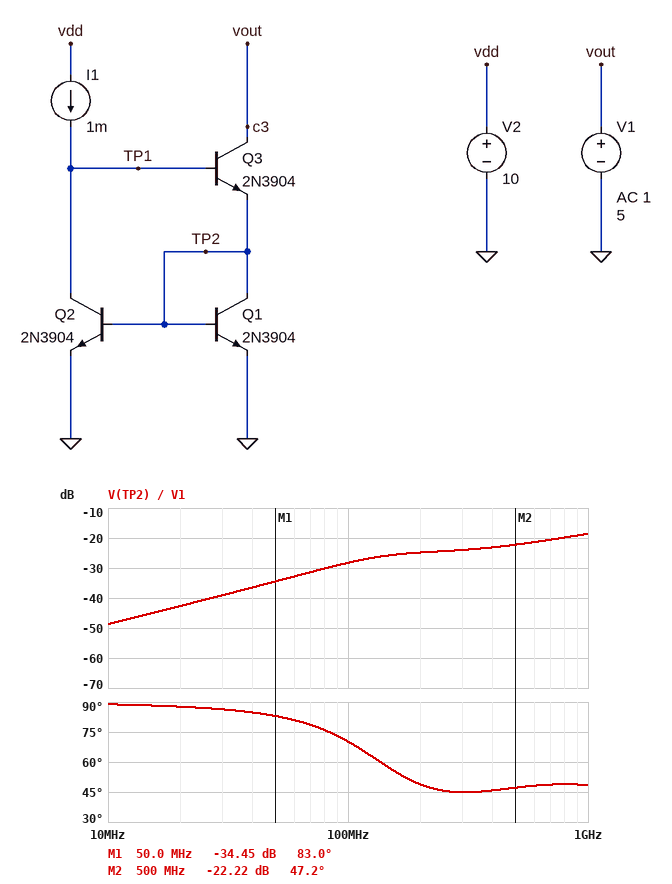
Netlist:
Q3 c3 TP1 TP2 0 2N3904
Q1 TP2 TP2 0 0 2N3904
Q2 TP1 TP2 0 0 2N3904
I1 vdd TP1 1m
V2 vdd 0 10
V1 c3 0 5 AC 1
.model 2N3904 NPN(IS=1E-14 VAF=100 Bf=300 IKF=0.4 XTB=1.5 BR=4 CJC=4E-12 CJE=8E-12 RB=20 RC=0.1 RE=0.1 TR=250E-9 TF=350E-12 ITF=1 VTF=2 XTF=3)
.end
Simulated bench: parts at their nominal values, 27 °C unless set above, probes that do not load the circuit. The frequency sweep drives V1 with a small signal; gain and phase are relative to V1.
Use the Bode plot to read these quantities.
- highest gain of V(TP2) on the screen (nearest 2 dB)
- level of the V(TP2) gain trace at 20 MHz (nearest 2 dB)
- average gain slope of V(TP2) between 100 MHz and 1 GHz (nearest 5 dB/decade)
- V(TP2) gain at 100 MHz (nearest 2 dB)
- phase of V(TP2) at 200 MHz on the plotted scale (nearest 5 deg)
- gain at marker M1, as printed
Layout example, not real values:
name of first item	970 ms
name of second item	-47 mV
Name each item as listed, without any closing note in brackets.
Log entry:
highest gain of V(TP2) on the screen	-18 dB
level of the V(TP2) gain trace at 20 MHz	-42 dB
average gain slope of V(TP2) between 100 MHz and 1 GHz	10 dB/decade
V(TP2) gain at 100 MHz	-28 dB
phase of V(TP2) at 200 MHz on the plotted scale	50 deg
gain at marker M1, as printed	-34.45 dB
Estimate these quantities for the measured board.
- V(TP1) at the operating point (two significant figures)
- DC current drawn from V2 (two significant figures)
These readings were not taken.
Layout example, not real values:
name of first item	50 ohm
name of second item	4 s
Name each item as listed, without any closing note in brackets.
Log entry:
V(TP1) at the operating point	1.3 V
DC current drawn from V2	1.0 mA
